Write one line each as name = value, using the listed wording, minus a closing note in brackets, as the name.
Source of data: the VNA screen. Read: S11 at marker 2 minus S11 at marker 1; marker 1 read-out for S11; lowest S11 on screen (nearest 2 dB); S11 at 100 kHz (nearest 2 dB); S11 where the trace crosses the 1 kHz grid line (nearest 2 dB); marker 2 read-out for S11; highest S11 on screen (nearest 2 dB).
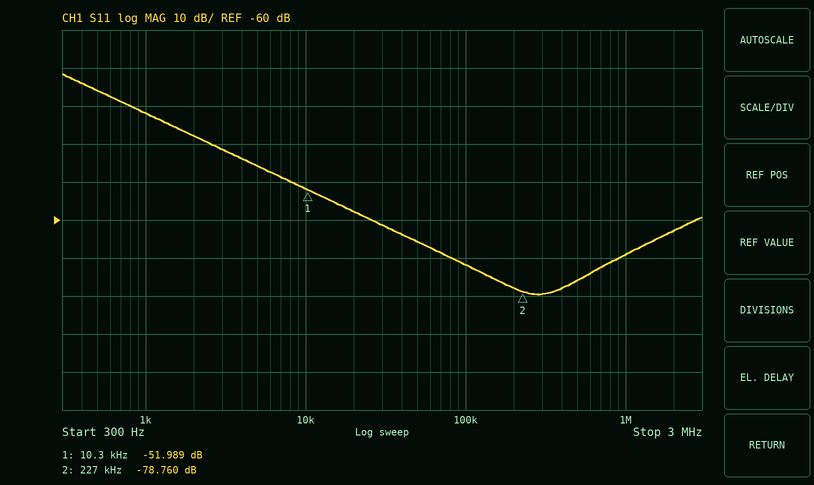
S11 at marker 2 minus S11 at marker 1 = -26.771 dB
marker 1 read-out for S11 = -51.989 dB
lowest S11 on screen = -80 dB
S11 at 100 kHz = -72 dB
S11 where the trace crosses the 1 kHz grid line = -32 dB
marker 2 read-out for S11 = -78.760 dB
highest S11 on screen = -22 dB
